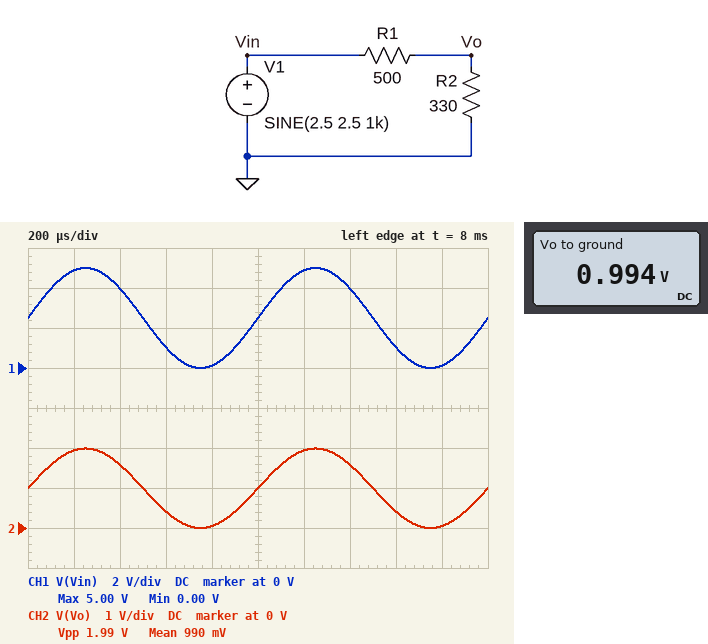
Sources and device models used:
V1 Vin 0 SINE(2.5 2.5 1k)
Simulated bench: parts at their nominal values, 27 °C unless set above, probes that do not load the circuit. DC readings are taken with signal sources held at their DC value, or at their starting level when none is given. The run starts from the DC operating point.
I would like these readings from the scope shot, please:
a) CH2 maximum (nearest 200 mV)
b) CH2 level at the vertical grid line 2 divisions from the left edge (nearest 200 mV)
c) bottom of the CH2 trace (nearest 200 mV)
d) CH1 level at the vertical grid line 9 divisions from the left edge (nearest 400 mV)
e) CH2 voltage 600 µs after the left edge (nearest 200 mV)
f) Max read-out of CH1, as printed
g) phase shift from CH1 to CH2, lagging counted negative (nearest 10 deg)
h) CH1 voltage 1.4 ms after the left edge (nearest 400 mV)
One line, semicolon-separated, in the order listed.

2.0 V; 1.6 V; 0 V; 0 V; 400 mV; 5.00 V; 0 deg; 4.0 V
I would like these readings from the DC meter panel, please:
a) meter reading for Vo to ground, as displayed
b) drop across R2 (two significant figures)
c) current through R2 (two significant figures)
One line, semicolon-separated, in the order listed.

0.994 V; 990 mV; 3.0 mA
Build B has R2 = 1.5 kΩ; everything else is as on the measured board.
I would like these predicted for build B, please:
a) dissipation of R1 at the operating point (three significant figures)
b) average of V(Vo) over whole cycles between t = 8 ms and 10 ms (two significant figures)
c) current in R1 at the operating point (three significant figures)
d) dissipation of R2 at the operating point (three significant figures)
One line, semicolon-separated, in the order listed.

781 µW; 1.9 V; 1.25 mA; 2.34 mW
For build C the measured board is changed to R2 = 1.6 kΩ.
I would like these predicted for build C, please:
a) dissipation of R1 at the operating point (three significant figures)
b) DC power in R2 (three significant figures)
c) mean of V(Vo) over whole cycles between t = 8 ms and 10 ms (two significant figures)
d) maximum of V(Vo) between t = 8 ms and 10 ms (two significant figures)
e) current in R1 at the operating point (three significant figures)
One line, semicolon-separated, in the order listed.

709 µW; 2.27 mW; 1.9 V; 3.8 V; 1.19 mA
